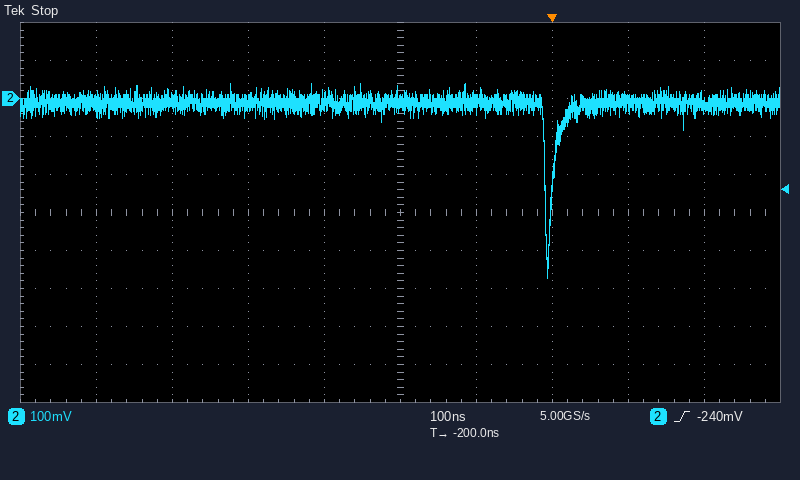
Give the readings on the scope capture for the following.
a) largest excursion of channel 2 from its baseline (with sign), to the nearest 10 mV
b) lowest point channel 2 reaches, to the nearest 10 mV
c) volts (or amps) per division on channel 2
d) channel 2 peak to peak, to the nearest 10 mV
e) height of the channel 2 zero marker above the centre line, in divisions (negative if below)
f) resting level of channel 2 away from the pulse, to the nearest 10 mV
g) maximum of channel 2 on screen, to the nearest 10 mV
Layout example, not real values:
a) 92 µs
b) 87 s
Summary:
a) -460 mV
b) -470 mV
c) 100 mV
d) 510 mV
e) +3.0 div
f) -10 mV
g) 40 mV
